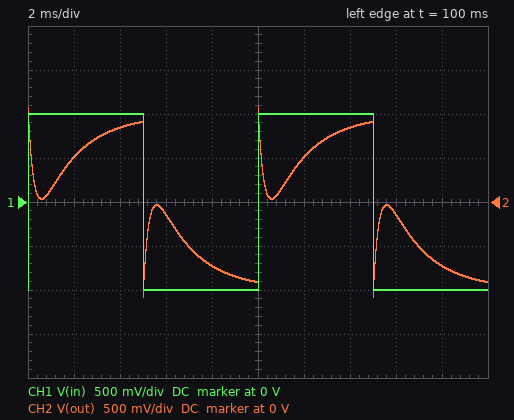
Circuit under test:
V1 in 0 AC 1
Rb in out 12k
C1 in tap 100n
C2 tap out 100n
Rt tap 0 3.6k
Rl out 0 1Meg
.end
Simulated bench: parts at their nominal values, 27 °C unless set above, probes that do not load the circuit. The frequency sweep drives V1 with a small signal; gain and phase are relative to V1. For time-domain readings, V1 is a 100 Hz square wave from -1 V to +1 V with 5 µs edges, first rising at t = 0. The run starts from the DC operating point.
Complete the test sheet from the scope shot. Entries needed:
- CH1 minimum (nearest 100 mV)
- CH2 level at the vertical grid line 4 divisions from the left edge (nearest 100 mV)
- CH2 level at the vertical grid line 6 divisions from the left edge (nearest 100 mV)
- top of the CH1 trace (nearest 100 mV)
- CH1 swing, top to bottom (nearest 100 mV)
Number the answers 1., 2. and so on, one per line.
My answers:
1. -1.0 V
2. -700 mV
3. 500 mV
4. 1.0 V
5. 2.0 V
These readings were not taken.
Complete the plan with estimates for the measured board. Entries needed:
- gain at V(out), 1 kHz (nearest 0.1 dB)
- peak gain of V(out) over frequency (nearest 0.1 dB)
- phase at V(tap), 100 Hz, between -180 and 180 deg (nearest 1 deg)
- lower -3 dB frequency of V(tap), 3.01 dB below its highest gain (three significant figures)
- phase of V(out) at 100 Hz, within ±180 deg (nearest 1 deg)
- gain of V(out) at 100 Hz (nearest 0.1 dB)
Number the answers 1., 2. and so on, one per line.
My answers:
1. -1.6 dB
2. 0 dB
3. 55 deg
4. 507 Hz
5. -27 deg
6. -3.9 dB
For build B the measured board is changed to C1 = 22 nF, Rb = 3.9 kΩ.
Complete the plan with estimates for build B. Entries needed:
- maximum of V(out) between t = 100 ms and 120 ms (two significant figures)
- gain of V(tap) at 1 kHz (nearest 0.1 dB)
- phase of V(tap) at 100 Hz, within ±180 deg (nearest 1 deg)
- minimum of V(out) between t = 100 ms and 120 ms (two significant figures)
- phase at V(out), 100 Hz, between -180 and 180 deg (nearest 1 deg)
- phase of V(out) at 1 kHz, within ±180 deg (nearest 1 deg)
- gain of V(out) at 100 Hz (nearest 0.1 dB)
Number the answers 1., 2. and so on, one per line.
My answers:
1. 990 mV
2. -4.8 dB
3. 65 deg
4. -990 mV
5. -12 deg
6. 2 deg
7. -0.8 dB
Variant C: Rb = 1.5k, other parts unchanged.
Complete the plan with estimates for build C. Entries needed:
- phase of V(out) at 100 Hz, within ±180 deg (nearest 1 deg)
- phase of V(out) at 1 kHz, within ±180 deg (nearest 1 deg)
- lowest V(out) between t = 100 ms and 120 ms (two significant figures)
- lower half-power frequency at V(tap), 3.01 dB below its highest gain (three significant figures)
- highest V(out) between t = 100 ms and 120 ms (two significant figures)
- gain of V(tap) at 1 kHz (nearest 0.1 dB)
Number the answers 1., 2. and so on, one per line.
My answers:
1. -4 deg
2. 2 deg
3. -1.0 V
4. 254 Hz
5. 1.0 V
6. -1.0 dB
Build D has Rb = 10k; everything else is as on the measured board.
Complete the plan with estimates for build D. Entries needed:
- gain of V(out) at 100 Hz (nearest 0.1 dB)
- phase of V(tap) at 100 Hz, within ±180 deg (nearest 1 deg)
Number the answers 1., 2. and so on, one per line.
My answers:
1. -3.1 dB
2. 56 deg
